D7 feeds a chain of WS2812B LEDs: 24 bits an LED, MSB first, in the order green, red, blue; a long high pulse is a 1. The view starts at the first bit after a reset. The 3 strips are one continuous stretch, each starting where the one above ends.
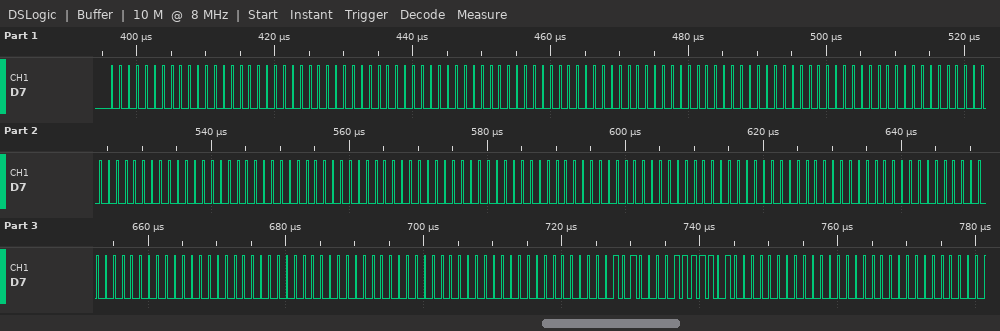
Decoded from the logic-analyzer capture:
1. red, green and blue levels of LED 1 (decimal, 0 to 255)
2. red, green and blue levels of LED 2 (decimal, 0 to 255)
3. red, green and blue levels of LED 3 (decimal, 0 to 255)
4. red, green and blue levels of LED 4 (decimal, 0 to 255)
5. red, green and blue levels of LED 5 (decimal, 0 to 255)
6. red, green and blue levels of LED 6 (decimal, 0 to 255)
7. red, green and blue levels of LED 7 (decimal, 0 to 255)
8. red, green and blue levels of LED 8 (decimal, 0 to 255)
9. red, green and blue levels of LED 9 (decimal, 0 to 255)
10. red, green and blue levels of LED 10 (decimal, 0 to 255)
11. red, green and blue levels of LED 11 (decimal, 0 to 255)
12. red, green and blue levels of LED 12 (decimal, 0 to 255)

0, 0, 0
0, 0, 0
0, 0, 0
0, 0, 0
0, 0, 0
0, 0, 0
0, 0, 0
0, 0, 0
0, 0, 0
0, 0, 0
0, 0, 0
250, 80, 0
